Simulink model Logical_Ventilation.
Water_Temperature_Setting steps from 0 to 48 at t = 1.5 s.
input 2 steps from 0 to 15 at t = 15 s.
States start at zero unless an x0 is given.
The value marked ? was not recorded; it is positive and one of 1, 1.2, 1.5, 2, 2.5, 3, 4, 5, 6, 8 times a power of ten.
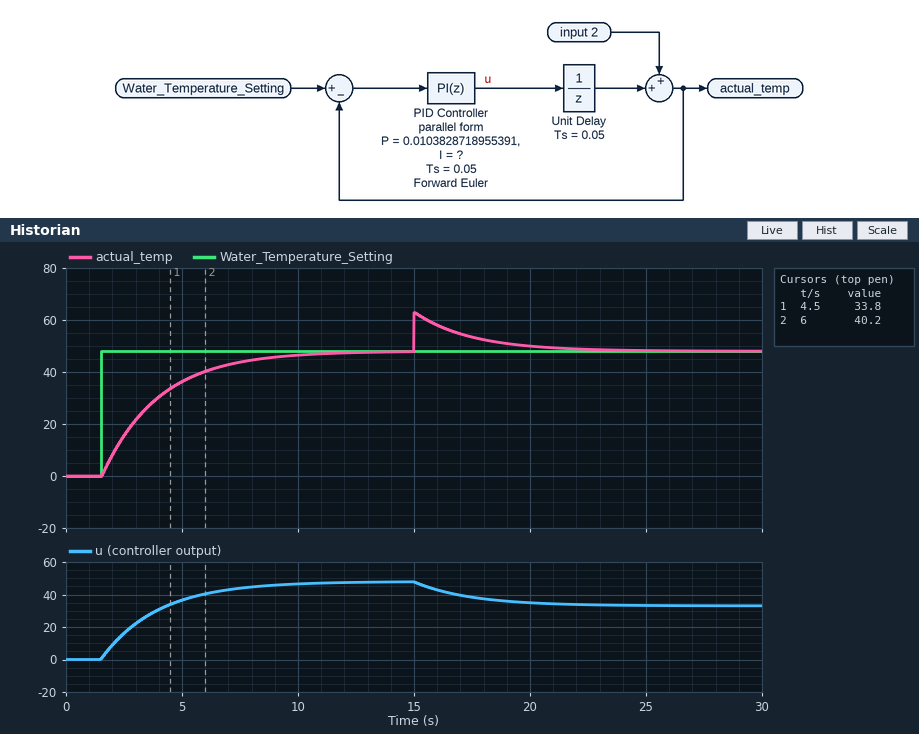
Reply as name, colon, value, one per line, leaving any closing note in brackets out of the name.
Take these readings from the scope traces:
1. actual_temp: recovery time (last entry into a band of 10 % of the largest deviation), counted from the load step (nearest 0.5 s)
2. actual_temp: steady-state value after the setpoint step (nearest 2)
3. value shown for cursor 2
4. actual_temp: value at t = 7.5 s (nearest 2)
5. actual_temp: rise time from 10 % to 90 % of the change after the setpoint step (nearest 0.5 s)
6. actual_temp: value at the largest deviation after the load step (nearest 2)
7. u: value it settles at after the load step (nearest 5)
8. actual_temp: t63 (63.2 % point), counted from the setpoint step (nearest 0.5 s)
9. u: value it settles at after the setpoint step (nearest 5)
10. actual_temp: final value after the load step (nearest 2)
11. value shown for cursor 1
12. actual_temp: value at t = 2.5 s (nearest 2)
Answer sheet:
actual_temp: recovery time (last entry into a band of 10 % of the largest deviation), counted from the load step: 5.5 s
actual_temp: steady-state value after the setpoint step: 48
value shown for cursor 2: 40.2
actual_temp: value at t = 7.5 s: 44
actual_temp: rise time from 10 % to 90 % of the change after the setpoint step: 5.5 s
actual_temp: value at the largest deviation after the load step: 62
u: value it settles at after the load step: 35
actual_temp: t63 (63.2 % point), counted from the setpoint step: 2.5 s
u: value it settles at after the setpoint step: 50
actual_temp: final value after the load step: 48
value shown for cursor 1: 33.8
actual_temp: value at t = 2.5 s: 16
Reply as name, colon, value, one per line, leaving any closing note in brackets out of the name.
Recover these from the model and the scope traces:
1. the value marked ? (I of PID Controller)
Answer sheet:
the value marked ?: 0.4
